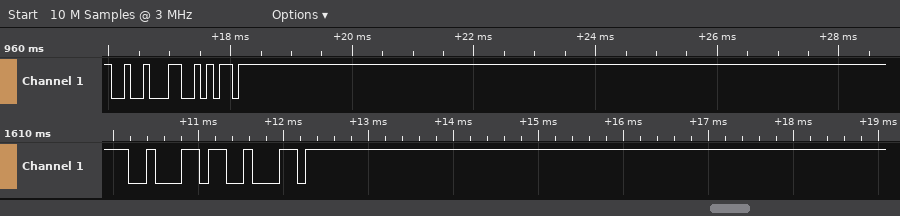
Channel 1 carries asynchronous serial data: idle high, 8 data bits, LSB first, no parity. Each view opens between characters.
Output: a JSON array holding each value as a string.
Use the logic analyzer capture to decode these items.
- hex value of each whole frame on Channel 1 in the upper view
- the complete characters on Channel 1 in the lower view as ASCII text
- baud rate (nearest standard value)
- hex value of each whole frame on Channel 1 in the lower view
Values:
["12, 6A", "\"bb\"", "9600 baud", "62, 62"]
